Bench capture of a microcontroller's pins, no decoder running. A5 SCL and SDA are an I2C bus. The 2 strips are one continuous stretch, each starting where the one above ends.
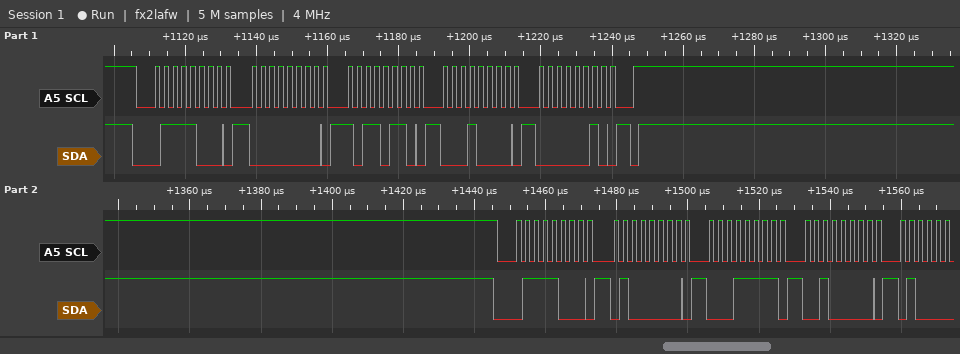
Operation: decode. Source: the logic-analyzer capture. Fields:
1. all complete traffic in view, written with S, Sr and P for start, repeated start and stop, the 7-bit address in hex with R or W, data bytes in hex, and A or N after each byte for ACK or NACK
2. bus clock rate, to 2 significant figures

S 3CW A 00 A B6 A 10 A 02 A P S 3CW A 40 A 1F A 20 A
400 kHz
